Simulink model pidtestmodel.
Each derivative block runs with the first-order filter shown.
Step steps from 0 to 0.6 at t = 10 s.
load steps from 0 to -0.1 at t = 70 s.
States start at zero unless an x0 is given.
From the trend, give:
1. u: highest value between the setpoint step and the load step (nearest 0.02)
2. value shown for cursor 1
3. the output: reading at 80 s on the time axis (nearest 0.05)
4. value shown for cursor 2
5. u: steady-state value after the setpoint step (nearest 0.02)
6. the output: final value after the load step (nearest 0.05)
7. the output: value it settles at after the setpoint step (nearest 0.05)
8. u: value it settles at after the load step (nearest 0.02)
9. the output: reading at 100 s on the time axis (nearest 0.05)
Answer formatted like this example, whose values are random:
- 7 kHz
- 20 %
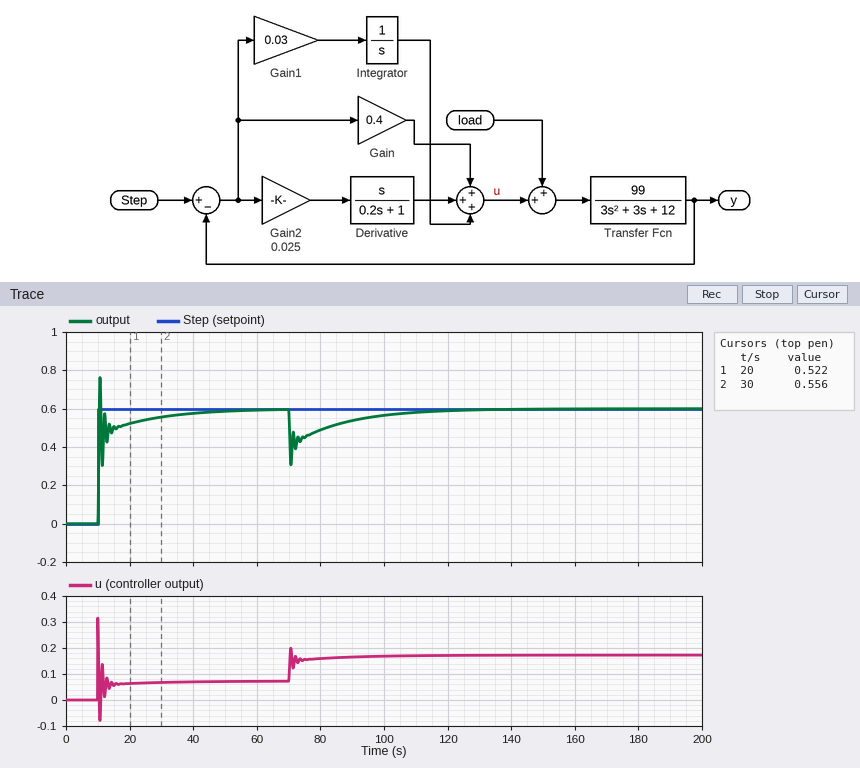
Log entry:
- 0.32
- 0.522
- 0.50
- 0.556
- 0.08
- 0.60
- 0.60
- 0.18
- 0.55
